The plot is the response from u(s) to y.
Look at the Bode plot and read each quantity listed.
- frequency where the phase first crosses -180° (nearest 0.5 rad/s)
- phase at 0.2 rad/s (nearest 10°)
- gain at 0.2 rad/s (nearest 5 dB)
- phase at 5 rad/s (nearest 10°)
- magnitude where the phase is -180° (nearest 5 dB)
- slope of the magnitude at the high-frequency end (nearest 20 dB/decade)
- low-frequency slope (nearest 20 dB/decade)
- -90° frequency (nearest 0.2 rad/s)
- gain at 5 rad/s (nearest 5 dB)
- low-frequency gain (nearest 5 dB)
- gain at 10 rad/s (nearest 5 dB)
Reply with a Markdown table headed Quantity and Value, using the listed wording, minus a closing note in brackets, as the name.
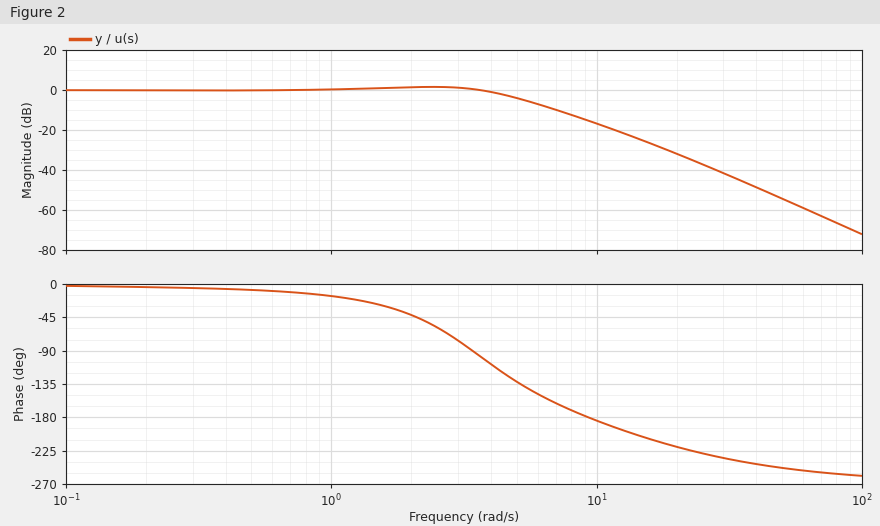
| Quantity | Value |
|---|---|
| frequency where the phase first crosses -180° | 9.5 rad/s |
| phase at 0.2 rad/s | 0° |
| gain at 0.2 rad/s | 0 dB |
| phase at 5 rad/s | -130° |
| magnitude where the phase is -180° | -15 dB |
| slope of the magnitude at the high-frequency end | -60 dB/decade |
| low-frequency slope | 0 dB/decade |
| -90° frequency | 3.4 rad/s |
| gain at 5 rad/s | -5 dB |
| low-frequency gain | 0 dB |
| gain at 10 rad/s | -15 dB |
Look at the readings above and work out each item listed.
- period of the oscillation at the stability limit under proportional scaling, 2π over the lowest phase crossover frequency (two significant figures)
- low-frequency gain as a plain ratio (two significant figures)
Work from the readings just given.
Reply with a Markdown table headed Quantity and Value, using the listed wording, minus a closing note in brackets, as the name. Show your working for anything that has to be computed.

| Quantity | Value |
|---|---|
| period of the oscillation at the stability limit under proportional scaling, 2π over the lowest phase crossover frequency | 2π / 9.5 = 0.66 s |
| low-frequency gain as a plain ratio | 10^(0 / 20) = 1.0 |
